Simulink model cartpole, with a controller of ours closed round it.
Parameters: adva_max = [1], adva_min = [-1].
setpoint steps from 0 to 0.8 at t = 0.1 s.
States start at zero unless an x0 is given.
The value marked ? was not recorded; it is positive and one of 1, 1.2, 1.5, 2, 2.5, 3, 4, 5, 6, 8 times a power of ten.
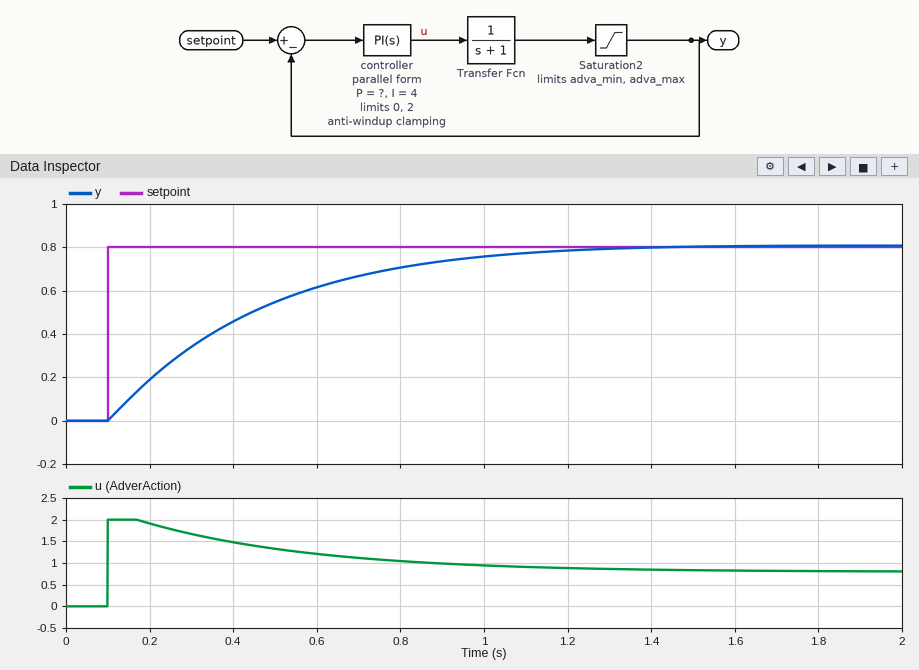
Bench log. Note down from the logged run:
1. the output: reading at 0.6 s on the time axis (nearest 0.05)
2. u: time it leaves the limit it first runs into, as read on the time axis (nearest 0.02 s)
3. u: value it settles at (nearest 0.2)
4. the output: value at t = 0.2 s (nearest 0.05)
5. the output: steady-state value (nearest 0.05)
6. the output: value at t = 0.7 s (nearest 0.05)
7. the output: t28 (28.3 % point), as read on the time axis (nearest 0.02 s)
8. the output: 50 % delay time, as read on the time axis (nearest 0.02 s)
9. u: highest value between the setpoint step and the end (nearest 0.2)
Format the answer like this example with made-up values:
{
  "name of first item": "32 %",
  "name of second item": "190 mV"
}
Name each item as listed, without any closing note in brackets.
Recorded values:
{
  "the output: reading at 0.6 s on the time axis": "0.60",
  "u: time it leaves the limit it first runs into, as read on the time axis": "0.18 s",
  "u: value it settles at": "0.8",
  "the output: value at t = 0.2 s": "0.20",
  "the output: steady-state value": "0.80",
  "the output: value at t = 0.7 s": "0.65",
  "the output: t28 (28.3 % point), as read on the time axis": "0.22 s",
  "the output: 50 % delay time, as read on the time axis": "0.34 s",
  "u: highest value between the setpoint step and the end": "2.0"
}
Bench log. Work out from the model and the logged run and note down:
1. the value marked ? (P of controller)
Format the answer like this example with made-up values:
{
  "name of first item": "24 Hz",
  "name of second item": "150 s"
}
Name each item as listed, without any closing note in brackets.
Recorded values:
{
  "the value marked ?": "3"
}
